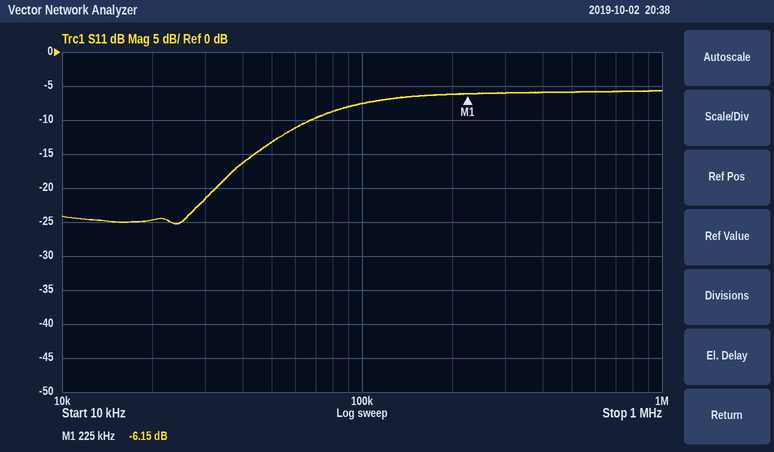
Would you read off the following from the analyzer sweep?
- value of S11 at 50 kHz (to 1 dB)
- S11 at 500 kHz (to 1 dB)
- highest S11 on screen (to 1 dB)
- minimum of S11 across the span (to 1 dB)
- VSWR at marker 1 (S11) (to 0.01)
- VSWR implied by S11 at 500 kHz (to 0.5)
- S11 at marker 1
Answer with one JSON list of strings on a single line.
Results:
["-13 dB", "-6 dB", "-6 dB", "-25 dB", "2.94", "3.0", "-6.15 dB"]
